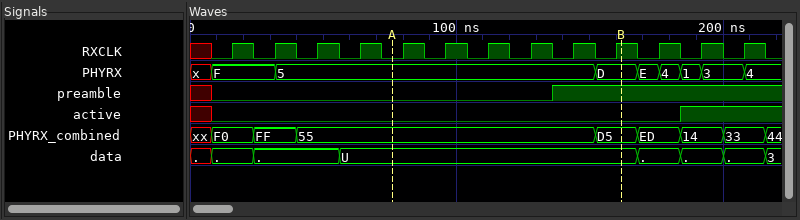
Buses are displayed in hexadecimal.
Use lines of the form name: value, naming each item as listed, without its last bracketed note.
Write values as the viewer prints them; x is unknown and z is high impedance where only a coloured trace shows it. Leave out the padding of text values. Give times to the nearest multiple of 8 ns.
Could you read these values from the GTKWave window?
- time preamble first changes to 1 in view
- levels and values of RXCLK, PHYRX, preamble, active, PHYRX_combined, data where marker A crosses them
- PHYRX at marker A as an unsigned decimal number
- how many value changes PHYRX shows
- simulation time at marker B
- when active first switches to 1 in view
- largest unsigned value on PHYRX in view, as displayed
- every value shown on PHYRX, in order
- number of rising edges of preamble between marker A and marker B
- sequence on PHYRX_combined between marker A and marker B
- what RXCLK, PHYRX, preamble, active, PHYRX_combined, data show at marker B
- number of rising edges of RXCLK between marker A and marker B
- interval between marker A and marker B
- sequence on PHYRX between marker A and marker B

time preamble first changes to 1 in view: 136 ns
levels and values of RXCLK, PHYRX, preamble, active, PHYRX_combined, data where marker A crosses them: RXCLK=0, PHYRX=5, preamble=0, active=0, PHYRX_combined=55, data=U
PHYRX at marker A as an unsigned decimal number: 5
how many value changes PHYRX shows: 8
simulation time at marker B: 160 ns
when active first switches to 1 in view: 184 ns
largest unsigned value on PHYRX in view, as displayed: F
every value shown on PHYRX, in order: x, F, 5, D, E, 4, 1, 3, 4
number of rising edges of preamble between marker A and marker B: 1
sequence on PHYRX_combined between marker A and marker B: 55, D5
what RXCLK, PHYRX, preamble, active, PHYRX_combined, data show at marker B: RXCLK=1, PHYRX=D, preamble=1, active=0, PHYRX_combined=D5, data=U
number of rising edges of RXCLK between marker A and marker B: 6
interval between marker A and marker B: 88 ns
sequence on PHYRX between marker A and marker B: 5, D
